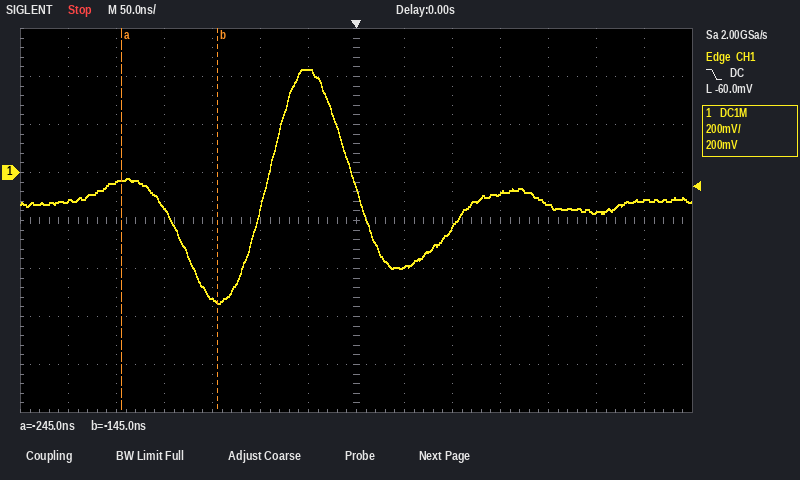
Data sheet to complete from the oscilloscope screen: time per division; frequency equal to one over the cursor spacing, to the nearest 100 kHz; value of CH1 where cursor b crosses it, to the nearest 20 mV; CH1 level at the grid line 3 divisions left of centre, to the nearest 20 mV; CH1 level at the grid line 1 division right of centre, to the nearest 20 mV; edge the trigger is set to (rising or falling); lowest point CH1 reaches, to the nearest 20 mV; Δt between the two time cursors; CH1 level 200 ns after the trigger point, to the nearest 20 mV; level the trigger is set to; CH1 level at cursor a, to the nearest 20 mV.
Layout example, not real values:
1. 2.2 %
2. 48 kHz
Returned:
1. 50 ns
2. 10.0 MHz
3. -540 mV
4. -520 mV
5. -400 mV
6. falling
7. -540 mV
8. 100 ns
9. -140 mV
10. -60.0 mV
11. -40 mV
